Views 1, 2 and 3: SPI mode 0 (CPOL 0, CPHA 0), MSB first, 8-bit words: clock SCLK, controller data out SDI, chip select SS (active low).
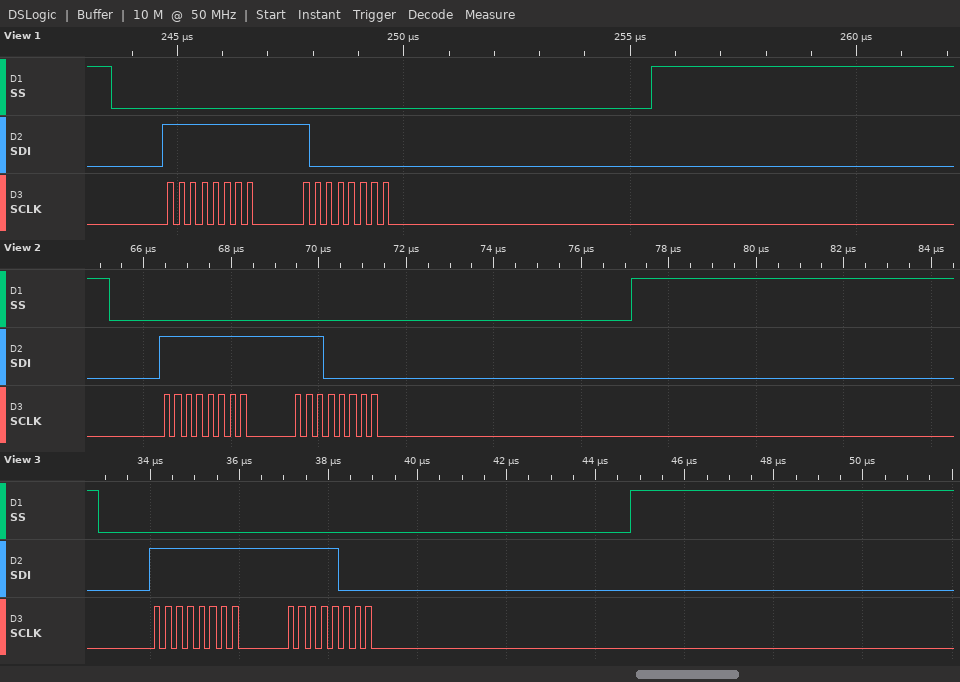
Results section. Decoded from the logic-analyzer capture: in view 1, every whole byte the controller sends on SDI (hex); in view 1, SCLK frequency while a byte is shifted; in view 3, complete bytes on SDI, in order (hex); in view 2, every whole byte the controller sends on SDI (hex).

FF 80
4 MHz
FF F8
FF E0
